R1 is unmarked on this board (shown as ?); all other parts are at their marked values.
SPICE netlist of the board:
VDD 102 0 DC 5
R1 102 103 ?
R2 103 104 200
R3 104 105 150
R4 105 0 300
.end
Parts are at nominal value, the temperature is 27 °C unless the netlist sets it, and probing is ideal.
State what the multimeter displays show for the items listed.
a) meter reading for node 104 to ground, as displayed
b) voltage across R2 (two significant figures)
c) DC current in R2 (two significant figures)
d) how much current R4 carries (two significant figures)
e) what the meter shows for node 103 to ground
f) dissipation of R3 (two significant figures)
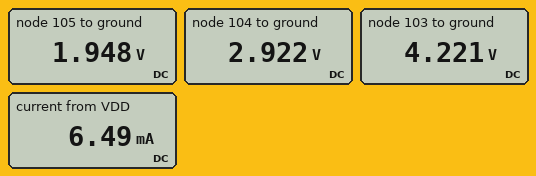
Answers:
2.922 V
1.3 V
6.5 mA
6.5 mA
4.221 V
6.3 mW
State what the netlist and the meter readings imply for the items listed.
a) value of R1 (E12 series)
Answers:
120 Ω
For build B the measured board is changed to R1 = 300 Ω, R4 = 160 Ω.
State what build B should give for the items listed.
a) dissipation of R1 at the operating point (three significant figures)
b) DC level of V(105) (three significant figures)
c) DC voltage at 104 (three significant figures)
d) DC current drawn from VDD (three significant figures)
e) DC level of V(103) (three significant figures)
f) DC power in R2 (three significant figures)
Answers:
11.4 mW
988 mV
1.91 V
6.17 mA
3.15 V
7.62 mW
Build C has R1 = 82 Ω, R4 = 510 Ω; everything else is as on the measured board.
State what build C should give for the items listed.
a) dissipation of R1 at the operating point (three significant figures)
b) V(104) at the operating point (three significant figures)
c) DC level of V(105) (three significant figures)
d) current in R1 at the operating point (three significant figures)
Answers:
2.31 mW
3.50 V
2.71 V
5.31 mA
